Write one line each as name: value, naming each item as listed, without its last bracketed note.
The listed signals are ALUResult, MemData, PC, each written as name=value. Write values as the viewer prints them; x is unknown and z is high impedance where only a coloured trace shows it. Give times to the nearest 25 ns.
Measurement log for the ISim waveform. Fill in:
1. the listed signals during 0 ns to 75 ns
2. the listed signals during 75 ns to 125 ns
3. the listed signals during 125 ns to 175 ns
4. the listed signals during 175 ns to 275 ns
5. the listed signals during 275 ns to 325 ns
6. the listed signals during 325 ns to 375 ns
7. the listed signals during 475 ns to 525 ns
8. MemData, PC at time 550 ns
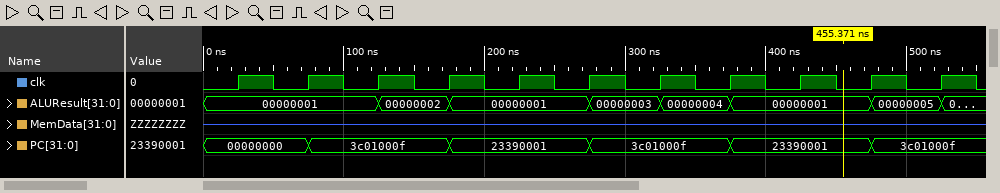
the listed signals during 0 ns to 75 ns: ALUResult=00000001, MemData=z, PC=00000000
the listed signals during 75 ns to 125 ns: ALUResult=00000001, MemData=z, PC=3c01000f
the listed signals during 125 ns to 175 ns: ALUResult=00000002, MemData=z, PC=3c01000f
the listed signals during 175 ns to 275 ns: ALUResult=00000001, MemData=z, PC=23390001
the listed signals during 275 ns to 325 ns: ALUResult=00000003, MemData=z, PC=3c01000f
the listed signals during 325 ns to 375 ns: ALUResult=00000004, MemData=z, PC=3c01000f
the listed signals during 475 ns to 525 ns: ALUResult=00000005, MemData=z, PC=3c01000f
MemData, PC at time 550 ns: MemData=z, PC=3c01000f
